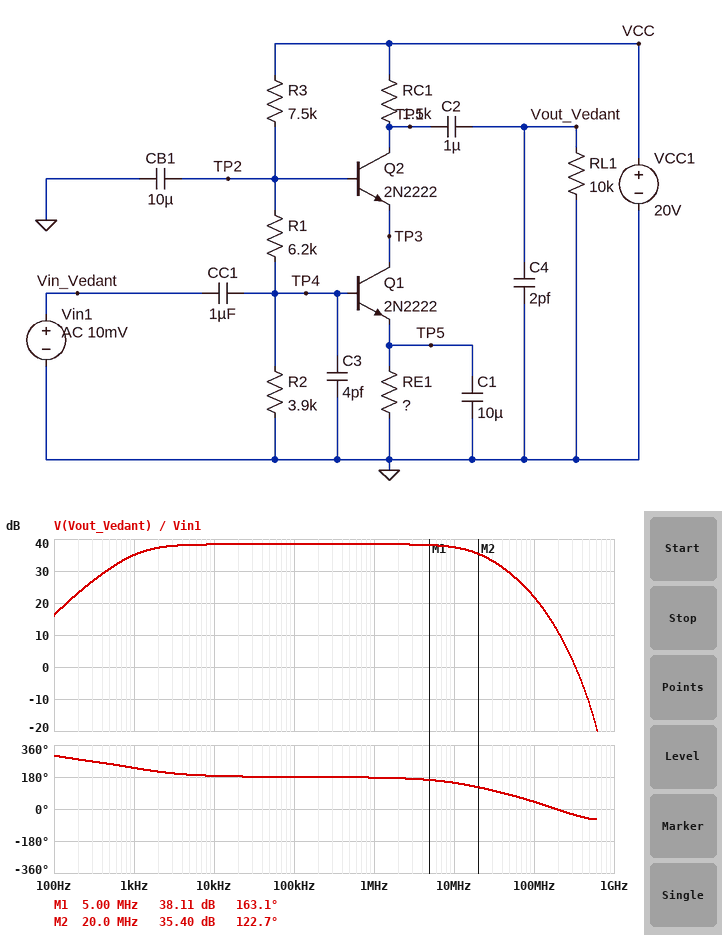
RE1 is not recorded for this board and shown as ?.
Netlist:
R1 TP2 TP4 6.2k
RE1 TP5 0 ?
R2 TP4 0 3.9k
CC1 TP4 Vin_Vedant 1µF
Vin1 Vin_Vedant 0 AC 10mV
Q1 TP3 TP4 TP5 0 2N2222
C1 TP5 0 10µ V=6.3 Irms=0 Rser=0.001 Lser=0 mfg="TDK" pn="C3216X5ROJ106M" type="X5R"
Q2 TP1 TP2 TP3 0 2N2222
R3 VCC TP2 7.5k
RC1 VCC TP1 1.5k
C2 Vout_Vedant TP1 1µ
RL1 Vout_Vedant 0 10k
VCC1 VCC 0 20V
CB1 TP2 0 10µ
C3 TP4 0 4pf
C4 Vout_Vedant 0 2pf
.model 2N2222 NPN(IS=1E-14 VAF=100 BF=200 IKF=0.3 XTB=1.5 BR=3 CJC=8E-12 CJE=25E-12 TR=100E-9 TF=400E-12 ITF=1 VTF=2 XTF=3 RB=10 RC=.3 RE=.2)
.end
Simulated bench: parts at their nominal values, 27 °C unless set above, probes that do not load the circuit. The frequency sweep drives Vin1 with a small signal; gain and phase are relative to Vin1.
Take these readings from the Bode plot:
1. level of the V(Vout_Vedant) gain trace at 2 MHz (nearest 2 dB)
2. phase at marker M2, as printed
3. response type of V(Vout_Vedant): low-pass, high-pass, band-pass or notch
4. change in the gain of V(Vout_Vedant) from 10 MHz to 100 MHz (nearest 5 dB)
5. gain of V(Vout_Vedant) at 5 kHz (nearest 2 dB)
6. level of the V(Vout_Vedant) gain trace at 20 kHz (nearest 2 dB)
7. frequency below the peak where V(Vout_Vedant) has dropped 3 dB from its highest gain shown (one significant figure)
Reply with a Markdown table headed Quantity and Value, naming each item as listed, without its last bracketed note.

| Quantity | Value |
|---|---|
| level of the V(Vout_Vedant) gain trace at 2 MHz | 38 dB |
| phase at marker M2, as printed | 122.7 deg |
| response type of V(Vout_Vedant): low-pass, high-pass, band-pass or notch | band-pass |
| change in the gain of V(Vout_Vedant) from 10 MHz to 100 MHz | -15 dB |
| gain of V(Vout_Vedant) at 5 kHz | 38 dB |
| level of the V(Vout_Vedant) gain trace at 20 kHz | 38 dB |
| frequency below the peak where V(Vout_Vedant) has dropped 3 dB from its highest gain shown | 1 kHz |
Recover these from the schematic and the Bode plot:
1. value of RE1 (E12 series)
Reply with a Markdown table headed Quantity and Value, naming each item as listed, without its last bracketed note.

| Quantity | Value |
|---|---|
| value of RE1 | 2.2 kΩ |
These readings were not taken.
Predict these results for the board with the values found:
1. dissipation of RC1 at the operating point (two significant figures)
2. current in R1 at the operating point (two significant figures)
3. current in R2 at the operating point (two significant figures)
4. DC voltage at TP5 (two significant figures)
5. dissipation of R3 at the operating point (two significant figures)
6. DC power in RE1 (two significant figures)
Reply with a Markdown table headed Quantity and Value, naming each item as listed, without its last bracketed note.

| Quantity | Value |
|---|---|
| dissipation of RC1 at the operating point | 4.2 mW |
| current in R1 at the operating point | 1.1 mA |
| current in R2 at the operating point | 1.1 mA |
| DC voltage at TP5 | 3.7 V |
| dissipation of R3 at the operating point | 9.8 mW |
| DC power in RE1 | 6.3 mW |
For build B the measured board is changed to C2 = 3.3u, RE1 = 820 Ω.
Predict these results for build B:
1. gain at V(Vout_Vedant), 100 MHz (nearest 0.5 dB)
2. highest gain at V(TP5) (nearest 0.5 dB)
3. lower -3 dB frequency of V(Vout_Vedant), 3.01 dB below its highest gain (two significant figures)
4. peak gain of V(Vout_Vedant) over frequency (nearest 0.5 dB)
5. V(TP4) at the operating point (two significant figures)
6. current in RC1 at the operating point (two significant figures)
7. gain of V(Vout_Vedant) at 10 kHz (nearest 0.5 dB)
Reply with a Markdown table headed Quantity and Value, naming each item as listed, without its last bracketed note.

| Quantity | Value |
|---|---|
| gain at V(Vout_Vedant), 100 MHz | 28.0 dB |
| highest gain at V(TP5) | -0.5 dB |
| lower -3 dB frequency of V(Vout_Vedant), 3.01 dB below its highest gain | 2.7 kHz |
| peak gain of V(Vout_Vedant) over frequency | 46.5 dB |
| V(TP4) at the operating point | 4.3 V |
| current in RC1 at the operating point | 4.4 mA |
| gain of V(Vout_Vedant) at 10 kHz | 46.0 dB |
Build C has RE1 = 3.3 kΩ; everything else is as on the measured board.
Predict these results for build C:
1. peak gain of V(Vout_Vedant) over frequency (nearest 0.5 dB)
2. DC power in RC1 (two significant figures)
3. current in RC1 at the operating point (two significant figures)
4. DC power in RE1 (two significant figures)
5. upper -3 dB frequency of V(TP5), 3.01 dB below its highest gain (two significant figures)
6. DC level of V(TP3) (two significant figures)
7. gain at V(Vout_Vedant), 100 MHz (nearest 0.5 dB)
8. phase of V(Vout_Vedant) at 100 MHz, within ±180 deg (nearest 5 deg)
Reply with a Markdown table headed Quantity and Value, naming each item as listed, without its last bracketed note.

| Quantity | Value |
|---|---|
| peak gain of V(Vout_Vedant) over frequency | 35.0 dB |
| DC power in RC1 | 1.9 mW |
| current in RC1 at the operating point | 1.1 mA |
| DC power in RE1 | 4.3 mW |
| upper -3 dB frequency of V(TP5), 3.01 dB below its highest gain | 850 Hz |
| DC level of V(TP3) | 11 V |
| gain at V(Vout_Vedant), 100 MHz | 18.0 dB |
| phase of V(Vout_Vedant) at 100 MHz, within ±180 deg | 35 deg |
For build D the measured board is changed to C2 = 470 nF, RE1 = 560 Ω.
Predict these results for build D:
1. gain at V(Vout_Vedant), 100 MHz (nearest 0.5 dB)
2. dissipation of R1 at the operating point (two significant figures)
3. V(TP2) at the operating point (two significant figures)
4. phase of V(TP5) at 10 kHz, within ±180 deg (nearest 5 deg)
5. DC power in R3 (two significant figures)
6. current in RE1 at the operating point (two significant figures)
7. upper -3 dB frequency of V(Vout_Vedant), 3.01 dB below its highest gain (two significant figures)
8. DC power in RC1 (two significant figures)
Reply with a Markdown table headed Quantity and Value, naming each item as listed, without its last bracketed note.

| Quantity | Value |
|---|---|
| gain at V(Vout_Vedant), 100 MHz | 4.0 dB |
| dissipation of R1 at the operating point | 7.8 mW |
| V(TP2) at the operating point | 11 V |
| phase of V(TP5) at 10 kHz, within ±180 deg | -70 deg |
| DC power in R3 | 10 mW |
| current in RE1 at the operating point | 6.3 mA |
| upper -3 dB frequency of V(Vout_Vedant), 3.01 dB below its highest gain | 1.0 MHz |
| DC power in RC1 | 59 mW |
